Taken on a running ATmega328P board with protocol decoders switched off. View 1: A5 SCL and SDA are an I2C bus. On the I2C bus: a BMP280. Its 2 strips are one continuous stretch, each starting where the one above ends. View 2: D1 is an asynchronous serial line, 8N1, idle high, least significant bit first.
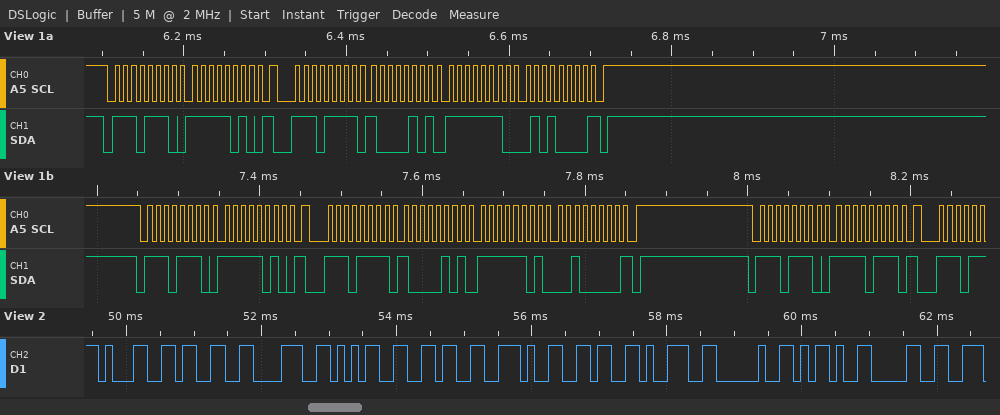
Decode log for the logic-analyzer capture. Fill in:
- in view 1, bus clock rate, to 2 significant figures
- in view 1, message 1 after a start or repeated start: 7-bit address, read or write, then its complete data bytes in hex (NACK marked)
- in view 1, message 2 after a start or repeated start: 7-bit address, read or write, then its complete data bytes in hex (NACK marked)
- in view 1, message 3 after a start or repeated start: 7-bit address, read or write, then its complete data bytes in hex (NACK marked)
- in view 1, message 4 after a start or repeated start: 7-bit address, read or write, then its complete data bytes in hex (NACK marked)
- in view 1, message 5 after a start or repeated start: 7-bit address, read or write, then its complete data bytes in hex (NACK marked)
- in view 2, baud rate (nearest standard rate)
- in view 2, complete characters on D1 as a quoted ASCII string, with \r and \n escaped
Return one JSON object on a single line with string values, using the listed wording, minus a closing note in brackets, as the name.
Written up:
{"in view 1, bus clock rate, to 2 significant figures": "100 kHz", "in view 1, message 1 after a start or repeated start: 7-bit address, read or write, then its complete data bytes in hex": "0x77 write: FA", "in view 1, message 2 after a start or repeated start: 7-bit address, read or write, then its complete data bytes in hex": "0x77 read: 85 FE 50 NACK", "in view 1, message 3 after a start or repeated start: 7-bit address, read or write, then its complete data bytes in hex": "0x77 write: FA", "in view 1, message 4 after a start or repeated start: 7-bit address, read or write, then its complete data bytes in hex": "0x77 read: 85 FD 20 NACK", "in view 1, message 5 after a start or repeated start: 7-bit address, read or write, then its complete data bytes in hex": "0x77 write: F7", "in view 2, baud rate": "9600 baud", "in view 2, complete characters on D1 as a quoted ASCII string, with \\r and \\n escaped": "\"13856.69 -0\""}
